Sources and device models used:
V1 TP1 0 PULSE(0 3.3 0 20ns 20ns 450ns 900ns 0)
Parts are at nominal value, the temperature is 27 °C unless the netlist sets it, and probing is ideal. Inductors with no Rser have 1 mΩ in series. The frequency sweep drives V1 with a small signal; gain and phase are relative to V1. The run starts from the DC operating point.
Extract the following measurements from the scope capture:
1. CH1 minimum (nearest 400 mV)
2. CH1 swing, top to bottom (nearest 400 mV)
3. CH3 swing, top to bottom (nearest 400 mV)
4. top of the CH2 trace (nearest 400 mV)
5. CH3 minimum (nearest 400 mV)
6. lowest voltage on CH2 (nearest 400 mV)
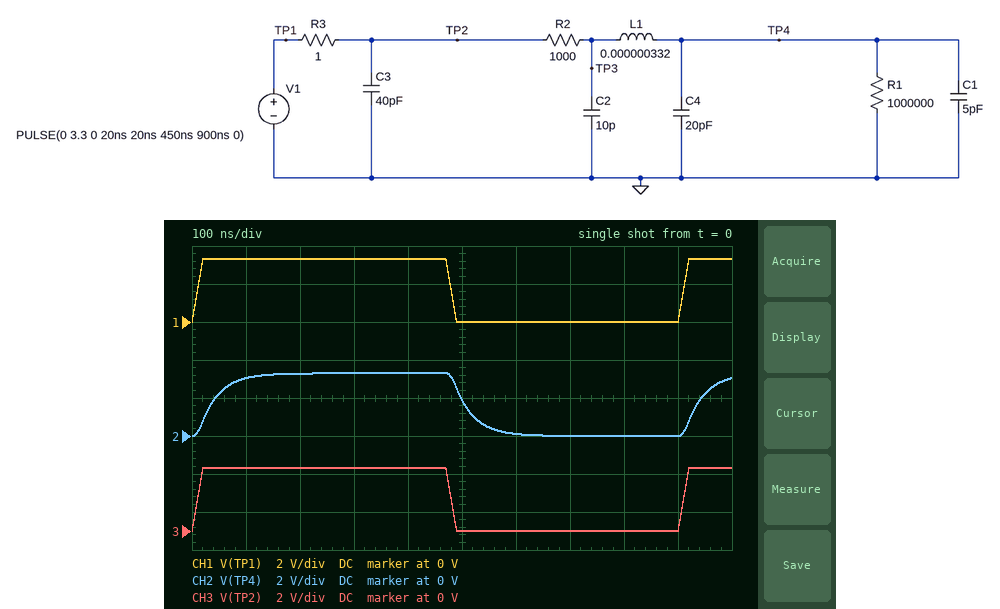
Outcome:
0 V
3.2 V
3.2 V
3.2 V
0 V
0 V
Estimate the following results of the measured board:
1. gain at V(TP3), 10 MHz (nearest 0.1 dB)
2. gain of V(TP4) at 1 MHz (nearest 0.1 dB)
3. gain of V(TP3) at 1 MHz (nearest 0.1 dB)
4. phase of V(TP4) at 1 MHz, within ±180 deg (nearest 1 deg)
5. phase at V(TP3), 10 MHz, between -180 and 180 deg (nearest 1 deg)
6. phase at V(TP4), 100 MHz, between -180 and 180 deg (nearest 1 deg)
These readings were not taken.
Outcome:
-7.8 dB
-0.2 dB
-0.2 dB
-12 deg
-66 deg
-150 deg
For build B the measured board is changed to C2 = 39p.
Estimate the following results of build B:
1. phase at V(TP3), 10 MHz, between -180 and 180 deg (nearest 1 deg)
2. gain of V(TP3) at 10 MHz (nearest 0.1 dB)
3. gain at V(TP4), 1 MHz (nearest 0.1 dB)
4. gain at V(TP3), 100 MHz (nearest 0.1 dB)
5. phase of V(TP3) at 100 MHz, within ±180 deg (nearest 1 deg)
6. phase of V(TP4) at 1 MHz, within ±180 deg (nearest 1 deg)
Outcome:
-76 deg
-12.5 dB
-0.7 dB
-24.9 dB
-88 deg
-22 deg
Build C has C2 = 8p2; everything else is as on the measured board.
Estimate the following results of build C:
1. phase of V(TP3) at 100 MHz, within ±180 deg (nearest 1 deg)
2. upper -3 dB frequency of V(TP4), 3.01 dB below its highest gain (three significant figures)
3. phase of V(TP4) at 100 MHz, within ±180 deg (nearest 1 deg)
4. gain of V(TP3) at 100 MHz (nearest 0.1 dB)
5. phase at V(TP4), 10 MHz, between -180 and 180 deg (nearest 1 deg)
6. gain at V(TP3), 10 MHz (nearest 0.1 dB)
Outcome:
59 deg
4.84 MHz
-121 deg
-6.1 dB
-65 deg
-7.5 dB
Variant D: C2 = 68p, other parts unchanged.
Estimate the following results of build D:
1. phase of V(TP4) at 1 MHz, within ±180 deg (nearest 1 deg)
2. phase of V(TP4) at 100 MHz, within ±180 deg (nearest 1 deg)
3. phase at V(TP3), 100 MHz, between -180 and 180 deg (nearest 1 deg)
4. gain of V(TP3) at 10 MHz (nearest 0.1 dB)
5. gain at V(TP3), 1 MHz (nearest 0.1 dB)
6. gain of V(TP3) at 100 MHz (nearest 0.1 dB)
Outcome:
-30 deg
90 deg
-90 deg
-15.5 dB
-1.3 dB
-31.1 dB
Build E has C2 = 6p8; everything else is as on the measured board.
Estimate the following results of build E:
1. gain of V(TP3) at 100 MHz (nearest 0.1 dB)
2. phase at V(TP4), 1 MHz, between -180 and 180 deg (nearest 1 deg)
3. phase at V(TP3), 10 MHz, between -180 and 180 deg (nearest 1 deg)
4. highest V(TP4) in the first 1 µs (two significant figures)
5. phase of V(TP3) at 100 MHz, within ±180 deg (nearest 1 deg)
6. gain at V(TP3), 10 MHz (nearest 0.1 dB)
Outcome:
-9.0 dB
-11 deg
-64 deg
3.3 V
68 deg
-7.2 dB
